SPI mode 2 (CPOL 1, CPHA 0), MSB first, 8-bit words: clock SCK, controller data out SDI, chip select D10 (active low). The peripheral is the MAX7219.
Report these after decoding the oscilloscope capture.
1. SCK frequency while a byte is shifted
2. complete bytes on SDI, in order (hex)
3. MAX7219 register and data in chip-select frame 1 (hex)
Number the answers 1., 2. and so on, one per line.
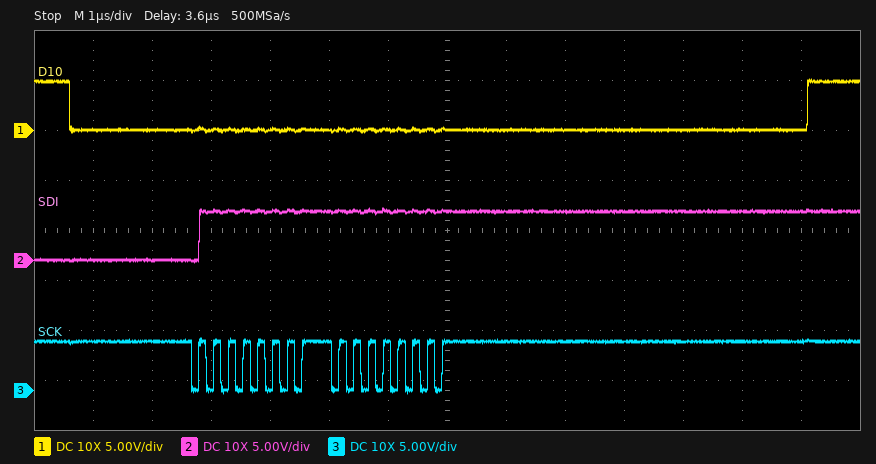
1. 4 MHz
2. 7F FF
3. register 0xF, data 0xFF
